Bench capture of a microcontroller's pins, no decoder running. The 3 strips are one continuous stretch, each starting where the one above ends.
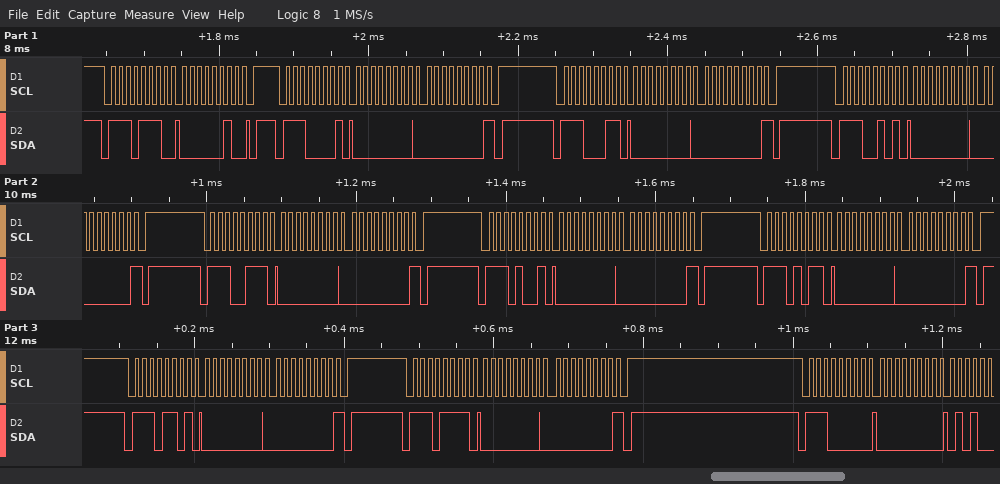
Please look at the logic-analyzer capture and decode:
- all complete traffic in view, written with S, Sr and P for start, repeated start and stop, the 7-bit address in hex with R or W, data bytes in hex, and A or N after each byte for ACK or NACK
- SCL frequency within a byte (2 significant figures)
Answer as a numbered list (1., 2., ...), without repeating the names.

1. S 77W A 02 A P S 70R A 00 A 00 N P S 71R A 00 A 00 N P S 72R A 00 A 00 N P S 73R A 00 A 00 N P S 74R A 00 A 00 N P S 75R A 00 A 00 N P S 76R A 00 A 00 N P S 77R A 00 A 00 N P S 70W A 00 A
2. 100 kHz
